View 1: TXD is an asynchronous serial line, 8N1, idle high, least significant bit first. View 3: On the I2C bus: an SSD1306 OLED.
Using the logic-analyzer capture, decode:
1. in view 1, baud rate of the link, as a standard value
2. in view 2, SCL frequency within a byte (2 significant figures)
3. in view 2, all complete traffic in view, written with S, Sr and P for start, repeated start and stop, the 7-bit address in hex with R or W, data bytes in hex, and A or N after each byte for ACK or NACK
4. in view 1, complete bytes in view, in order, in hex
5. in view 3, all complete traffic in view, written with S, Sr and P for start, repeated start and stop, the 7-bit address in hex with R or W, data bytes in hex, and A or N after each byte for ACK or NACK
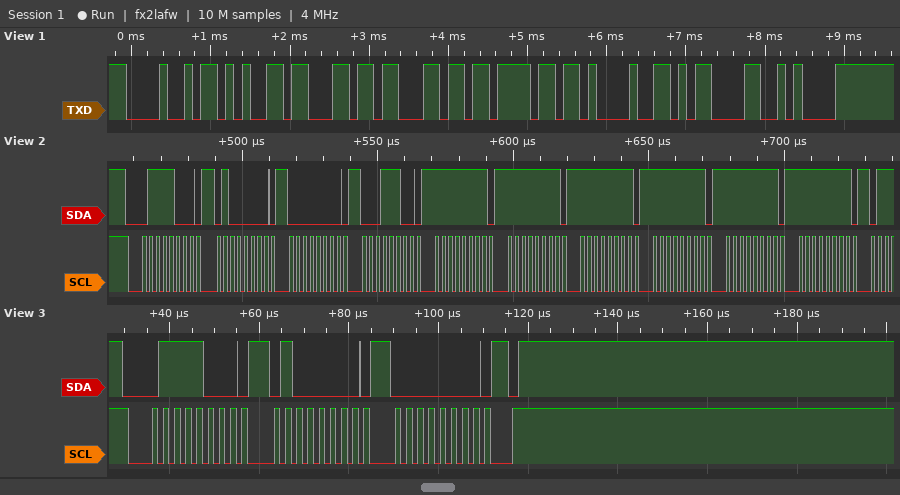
9600 baud
400 kHz
S 3CW A 40 A 00 A 1C A FF A FF A FF A FF A FF A FF A
48 65 6C 6C 6F 21 0D 0A
S 3CW A 40 A 00 A P
